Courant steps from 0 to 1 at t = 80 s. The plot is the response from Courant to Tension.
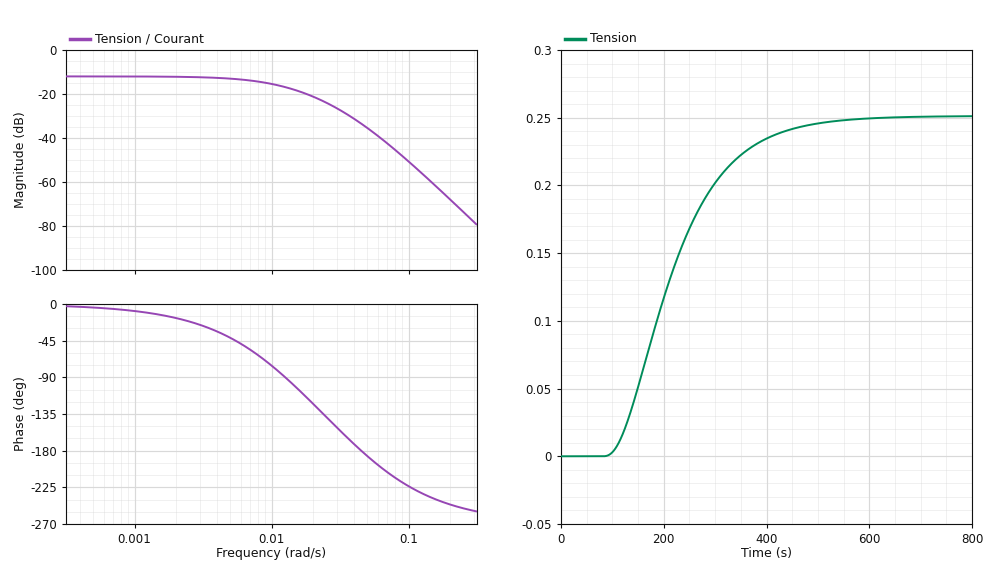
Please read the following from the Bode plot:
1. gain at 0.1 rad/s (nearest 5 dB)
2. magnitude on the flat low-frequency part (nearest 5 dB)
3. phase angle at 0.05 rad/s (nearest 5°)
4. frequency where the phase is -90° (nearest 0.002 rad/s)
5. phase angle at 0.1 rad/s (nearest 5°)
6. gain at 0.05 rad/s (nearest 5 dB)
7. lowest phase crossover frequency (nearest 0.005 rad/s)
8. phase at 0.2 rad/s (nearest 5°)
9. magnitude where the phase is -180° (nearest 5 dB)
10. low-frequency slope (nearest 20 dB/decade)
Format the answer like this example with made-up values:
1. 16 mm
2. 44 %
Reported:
1. -50 dB
2. -10 dB
3. -185°
4. 0.012 rad/s
5. -225°
6. -35 dB
7. 0.045 rad/s
8. -245°
9. -35 dB
10. 0 dB/decade
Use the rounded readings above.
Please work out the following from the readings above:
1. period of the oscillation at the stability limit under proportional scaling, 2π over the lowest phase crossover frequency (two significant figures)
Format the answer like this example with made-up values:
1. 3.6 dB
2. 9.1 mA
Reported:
1. 140 s
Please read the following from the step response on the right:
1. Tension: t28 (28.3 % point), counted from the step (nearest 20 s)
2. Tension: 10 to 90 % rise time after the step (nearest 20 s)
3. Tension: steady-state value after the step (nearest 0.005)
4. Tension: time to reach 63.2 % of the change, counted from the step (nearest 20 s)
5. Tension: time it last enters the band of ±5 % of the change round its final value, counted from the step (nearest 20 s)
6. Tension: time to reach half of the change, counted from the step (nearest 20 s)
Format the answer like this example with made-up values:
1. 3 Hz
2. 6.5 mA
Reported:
1. 80 s
2. 240 s
3. 0.250
4. 160 s
5. 340 s
6. 120 s
